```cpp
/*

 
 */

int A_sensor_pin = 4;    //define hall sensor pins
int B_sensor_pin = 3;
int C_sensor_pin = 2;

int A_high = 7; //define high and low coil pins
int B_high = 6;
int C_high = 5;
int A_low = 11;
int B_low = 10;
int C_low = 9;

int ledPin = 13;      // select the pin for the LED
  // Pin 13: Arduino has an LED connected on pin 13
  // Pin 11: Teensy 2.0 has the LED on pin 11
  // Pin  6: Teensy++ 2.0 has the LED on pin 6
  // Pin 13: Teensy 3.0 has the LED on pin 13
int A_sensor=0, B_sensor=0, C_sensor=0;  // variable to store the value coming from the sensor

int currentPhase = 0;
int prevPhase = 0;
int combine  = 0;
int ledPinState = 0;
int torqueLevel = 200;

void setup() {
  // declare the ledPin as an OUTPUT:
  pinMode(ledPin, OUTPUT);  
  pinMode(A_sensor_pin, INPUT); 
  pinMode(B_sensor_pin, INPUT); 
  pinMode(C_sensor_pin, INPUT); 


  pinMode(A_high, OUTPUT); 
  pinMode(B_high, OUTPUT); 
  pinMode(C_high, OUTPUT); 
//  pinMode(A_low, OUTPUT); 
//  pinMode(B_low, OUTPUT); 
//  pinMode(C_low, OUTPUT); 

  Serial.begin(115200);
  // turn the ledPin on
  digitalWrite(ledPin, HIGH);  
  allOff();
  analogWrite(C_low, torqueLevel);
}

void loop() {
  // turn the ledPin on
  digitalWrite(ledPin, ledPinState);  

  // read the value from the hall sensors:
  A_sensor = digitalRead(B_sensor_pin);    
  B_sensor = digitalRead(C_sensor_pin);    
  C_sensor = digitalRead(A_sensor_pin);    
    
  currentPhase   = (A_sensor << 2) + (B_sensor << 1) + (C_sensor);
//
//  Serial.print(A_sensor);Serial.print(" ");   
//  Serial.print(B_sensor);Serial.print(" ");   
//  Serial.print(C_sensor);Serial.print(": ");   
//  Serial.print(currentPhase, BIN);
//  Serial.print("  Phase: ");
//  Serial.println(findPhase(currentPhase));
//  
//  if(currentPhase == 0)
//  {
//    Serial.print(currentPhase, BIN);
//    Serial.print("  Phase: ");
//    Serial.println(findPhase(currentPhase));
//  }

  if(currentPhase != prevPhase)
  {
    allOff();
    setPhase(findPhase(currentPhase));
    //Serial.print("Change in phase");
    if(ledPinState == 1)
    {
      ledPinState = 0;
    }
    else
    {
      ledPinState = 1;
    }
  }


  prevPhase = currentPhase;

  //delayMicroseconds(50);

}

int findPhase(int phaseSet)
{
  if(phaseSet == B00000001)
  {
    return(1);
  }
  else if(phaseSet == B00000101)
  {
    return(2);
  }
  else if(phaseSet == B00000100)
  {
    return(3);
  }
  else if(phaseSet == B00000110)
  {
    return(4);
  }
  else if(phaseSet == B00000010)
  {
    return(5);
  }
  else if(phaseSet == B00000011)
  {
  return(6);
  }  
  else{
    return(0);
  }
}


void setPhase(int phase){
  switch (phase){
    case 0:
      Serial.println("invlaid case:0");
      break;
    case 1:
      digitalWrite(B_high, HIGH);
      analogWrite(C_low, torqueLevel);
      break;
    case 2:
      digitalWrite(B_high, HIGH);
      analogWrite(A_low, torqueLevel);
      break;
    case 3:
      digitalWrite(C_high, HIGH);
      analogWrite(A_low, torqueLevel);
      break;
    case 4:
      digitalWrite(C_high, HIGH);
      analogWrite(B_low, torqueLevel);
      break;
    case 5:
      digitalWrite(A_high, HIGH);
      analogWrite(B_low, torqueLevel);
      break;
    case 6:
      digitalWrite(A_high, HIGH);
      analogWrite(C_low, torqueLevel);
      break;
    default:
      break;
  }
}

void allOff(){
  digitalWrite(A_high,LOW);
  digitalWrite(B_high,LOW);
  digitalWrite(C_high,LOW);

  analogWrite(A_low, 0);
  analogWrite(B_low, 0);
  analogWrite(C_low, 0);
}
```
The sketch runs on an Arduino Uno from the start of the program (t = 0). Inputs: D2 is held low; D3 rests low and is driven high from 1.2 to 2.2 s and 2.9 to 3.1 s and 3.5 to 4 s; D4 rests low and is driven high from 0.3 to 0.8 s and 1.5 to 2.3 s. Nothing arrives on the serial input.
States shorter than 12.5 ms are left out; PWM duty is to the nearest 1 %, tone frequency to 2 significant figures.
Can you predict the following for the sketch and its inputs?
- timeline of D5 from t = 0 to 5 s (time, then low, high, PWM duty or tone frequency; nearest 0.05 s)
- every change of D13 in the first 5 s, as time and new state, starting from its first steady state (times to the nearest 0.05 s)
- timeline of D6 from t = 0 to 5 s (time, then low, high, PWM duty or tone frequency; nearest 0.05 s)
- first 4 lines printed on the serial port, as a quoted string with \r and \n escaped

0 s low; 1.2 s high; 1.5 s low; 2.9 s high; 3.1 s low; 3.5 s high; 4 s low
0 s low; 0.3 s high; 0.8 s low; 1.2 s high; 1.5 s low; 2.2 s high; 2.3 s low; 2.9 s high; 3.1 s low; 3.5 s high; 4 s low
0 s low; 0.3 s high; 0.8 s low; 1.5 s high; 2.3 s low
"invlaid case:0\r\ninvlaid case:0\r\ninvlaid case:0\r\ninvlaid case:0\r\n"
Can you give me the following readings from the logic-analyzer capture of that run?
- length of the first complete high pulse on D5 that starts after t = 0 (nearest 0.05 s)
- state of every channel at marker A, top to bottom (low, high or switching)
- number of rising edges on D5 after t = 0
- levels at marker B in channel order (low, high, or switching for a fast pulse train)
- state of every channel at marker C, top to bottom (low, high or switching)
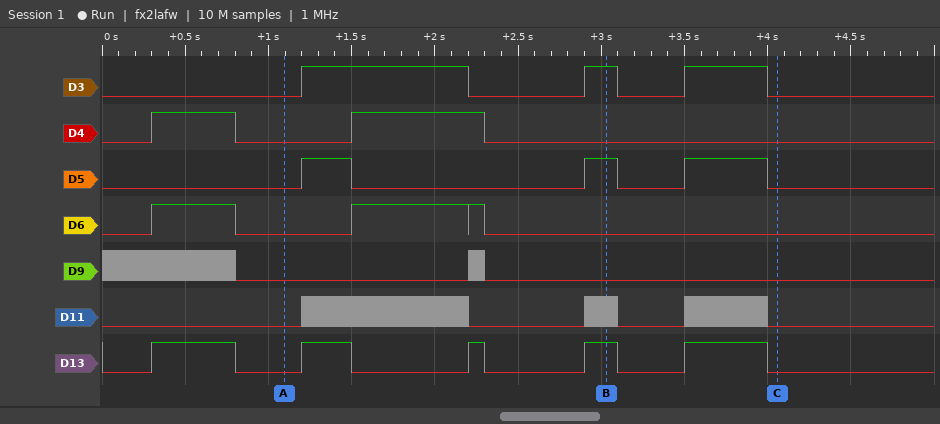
0.30 s
D3 low, D4 low, D5 low, D6 low, D9 low, D11 low, D13 low
3
D3 high, D4 low, D5 high, D6 low, D9 low, D11 switching, D13 high
D3 low, D4 low, D5 low, D6 low, D9 low, D11 low, D13 low
